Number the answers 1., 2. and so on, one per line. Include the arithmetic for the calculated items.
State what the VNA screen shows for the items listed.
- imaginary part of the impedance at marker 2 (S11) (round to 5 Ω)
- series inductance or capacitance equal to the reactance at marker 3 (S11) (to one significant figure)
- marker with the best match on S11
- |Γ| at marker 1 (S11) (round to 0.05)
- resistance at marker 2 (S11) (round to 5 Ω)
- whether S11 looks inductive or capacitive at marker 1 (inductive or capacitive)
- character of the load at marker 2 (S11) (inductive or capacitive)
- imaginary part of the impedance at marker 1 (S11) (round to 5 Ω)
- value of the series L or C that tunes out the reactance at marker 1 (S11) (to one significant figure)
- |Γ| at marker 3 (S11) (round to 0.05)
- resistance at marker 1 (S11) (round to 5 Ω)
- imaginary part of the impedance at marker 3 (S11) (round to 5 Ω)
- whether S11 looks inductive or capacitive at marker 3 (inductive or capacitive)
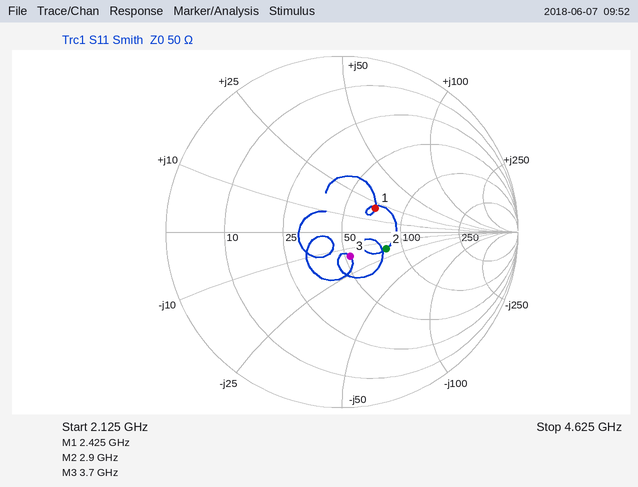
1. -15 Ω
2. C = 1/(2π × 3.7 GHz × 15 Ω) ≈ 3 pF
3. marker 3
4. 0.25
5. 80 Ω
6. inductive
7. capacitive
8. +20 Ω
9. C = 1/(2π × 2.425 GHz × 20 Ω) ≈ 3 pF
10. 0.15
11. 70 Ω
12. -15 Ω
13. capacitive
